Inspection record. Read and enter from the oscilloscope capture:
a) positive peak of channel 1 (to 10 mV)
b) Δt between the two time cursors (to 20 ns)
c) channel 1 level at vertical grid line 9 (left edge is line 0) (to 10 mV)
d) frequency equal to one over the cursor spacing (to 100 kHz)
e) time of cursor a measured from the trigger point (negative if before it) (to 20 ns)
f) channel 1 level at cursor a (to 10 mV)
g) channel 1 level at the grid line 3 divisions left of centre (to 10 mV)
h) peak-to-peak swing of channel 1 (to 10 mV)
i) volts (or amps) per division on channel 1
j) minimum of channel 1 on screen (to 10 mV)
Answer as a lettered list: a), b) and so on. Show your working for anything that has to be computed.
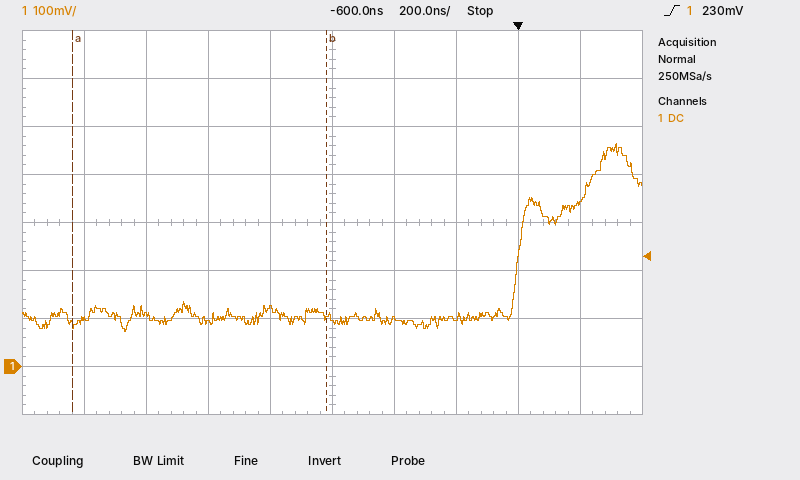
a) 460 mV
b) 820 ns
c) 340 mV
d) 1 / 820 ns ≈ 1.2 MHz
e) -1.44 µs
f) 90 mV
g) 110 mV
h) 460 mV − (70 mV) = 390 mV
i) 100 mV
j) 70 mV
